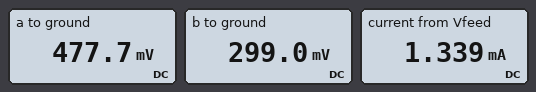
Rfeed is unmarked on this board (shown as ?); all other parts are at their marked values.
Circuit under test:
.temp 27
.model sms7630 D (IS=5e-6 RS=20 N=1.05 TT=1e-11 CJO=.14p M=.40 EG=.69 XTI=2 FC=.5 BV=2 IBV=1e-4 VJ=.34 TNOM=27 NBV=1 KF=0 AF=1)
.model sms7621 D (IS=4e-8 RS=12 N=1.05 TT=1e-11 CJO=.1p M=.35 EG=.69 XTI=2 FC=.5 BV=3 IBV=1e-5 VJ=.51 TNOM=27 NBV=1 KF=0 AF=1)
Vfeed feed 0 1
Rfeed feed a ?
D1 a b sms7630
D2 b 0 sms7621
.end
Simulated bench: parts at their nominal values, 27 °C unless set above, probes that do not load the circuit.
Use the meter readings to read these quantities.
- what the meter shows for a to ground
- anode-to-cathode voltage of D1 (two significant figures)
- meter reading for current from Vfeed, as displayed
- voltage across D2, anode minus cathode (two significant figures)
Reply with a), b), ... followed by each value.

a) 477.7 mV
b) 180 mV
c) 1.339 mA
d) 300 mV
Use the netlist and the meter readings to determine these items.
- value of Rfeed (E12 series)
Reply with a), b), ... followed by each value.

a) 390 Ω
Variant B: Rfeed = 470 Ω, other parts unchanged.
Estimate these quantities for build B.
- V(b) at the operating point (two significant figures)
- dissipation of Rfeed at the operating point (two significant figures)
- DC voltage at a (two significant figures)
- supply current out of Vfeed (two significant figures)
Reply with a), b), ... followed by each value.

a) 290 mV
b) 610 µW
c) 460 mV
d) 1.1 mA
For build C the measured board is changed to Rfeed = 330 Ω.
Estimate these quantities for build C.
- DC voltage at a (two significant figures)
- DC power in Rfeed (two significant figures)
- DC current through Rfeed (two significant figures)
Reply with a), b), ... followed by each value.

a) 490 mV
b) 780 µW
c) 1.5 mA
